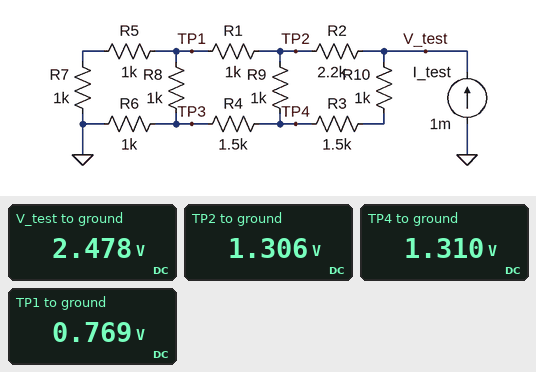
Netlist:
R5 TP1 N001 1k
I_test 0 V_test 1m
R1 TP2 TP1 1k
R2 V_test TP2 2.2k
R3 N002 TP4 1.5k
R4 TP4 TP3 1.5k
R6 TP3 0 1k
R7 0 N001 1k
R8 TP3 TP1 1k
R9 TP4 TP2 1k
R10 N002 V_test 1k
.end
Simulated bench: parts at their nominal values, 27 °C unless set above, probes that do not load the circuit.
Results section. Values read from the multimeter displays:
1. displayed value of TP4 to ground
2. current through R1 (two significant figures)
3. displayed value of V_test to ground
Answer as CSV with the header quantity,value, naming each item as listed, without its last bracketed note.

quantity,value
displayed value of TP4 to ground,1.310 V
current through R1,540 µA
displayed value of V_test to ground,2.478 V
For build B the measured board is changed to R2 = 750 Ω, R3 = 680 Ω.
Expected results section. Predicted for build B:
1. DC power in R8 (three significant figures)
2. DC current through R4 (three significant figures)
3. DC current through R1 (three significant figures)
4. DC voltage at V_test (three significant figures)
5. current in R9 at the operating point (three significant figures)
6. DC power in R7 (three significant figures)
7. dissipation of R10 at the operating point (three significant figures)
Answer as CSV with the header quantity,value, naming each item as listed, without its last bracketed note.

quantity,value
DC power in R8,30.4 µW
DC current through R4,434 µA
DC current through R1,566 µA
DC voltage at V_test,1.84 V
current in R9 at the operating point,88.9 µA
DC power in R7,153 µW
dissipation of R10 at the operating point,119 µW
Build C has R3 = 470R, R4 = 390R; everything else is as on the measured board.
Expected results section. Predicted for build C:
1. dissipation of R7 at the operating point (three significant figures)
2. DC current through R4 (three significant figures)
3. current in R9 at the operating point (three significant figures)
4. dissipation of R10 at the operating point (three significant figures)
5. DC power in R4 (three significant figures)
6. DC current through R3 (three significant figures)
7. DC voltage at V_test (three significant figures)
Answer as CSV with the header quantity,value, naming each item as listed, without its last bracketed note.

quantity,value
dissipation of R7 at the operating point,110 µW
DC current through R4,674 µA
current in R9 at the operating point,58.3 µA
dissipation of R10 at the operating point,379 µW
DC power in R4,177 µW
DC current through R3,615 µA
DC voltage at V_test,1.84 V
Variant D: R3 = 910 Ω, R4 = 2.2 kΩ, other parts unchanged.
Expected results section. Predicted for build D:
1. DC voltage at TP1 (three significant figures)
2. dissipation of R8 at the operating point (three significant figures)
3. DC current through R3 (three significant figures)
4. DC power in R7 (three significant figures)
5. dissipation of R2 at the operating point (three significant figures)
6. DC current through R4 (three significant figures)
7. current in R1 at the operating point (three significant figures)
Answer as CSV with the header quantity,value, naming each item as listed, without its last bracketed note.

quantity,value
DC voltage at TP1,797 mV
dissipation of R8 at the operating point,38.2 µW
DC current through R3,510 µA
DC power in R7,159 µW
dissipation of R2 at the operating point,528 µW
DC current through R4,406 µA
current in R1 at the operating point,594 µA
